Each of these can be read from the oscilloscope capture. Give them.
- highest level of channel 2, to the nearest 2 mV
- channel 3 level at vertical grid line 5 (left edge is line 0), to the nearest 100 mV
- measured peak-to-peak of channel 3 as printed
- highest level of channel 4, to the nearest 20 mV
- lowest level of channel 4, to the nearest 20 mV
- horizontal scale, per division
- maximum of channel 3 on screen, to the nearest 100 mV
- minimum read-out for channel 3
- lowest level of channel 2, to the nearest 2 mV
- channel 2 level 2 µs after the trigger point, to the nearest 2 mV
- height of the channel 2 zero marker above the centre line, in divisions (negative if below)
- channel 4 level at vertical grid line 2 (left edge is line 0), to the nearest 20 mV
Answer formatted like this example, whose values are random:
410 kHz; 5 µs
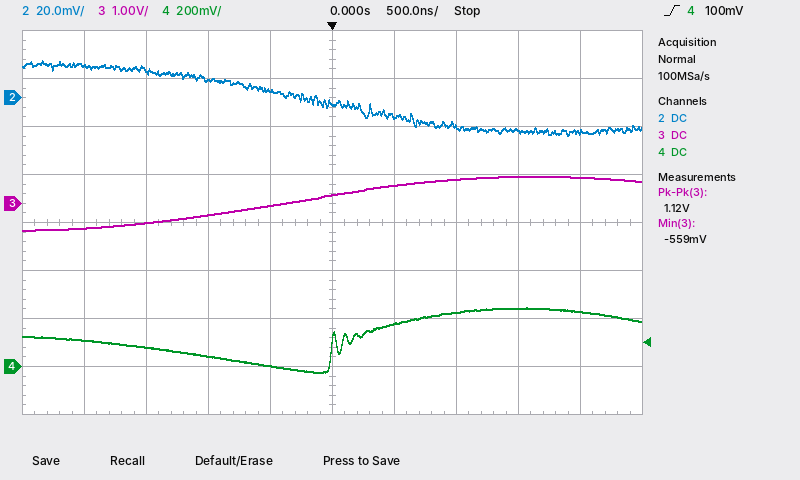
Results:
16 mV; 200 mV; 1.12 V; 240 mV; -20 mV; 500 ns; 600 mV; -559 mV; -16 mV; -14 mV; +2.6 div; 80 mV
